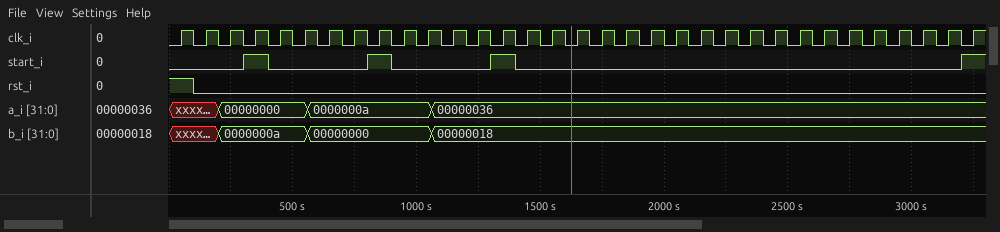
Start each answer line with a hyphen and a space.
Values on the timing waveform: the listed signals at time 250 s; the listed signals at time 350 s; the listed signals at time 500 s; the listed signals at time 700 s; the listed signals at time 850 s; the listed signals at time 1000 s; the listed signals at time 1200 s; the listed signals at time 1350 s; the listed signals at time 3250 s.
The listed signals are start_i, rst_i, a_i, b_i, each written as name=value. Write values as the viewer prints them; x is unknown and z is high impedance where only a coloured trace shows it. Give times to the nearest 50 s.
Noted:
- start_i=0, rst_i=0, a_i=00000000, b_i=0000000a
- start_i=1, rst_i=0, a_i=00000000, b_i=0000000a
- start_i=0, rst_i=0, a_i=00000000, b_i=0000000a
- start_i=0, rst_i=0, a_i=0000000a, b_i=00000000
- start_i=1, rst_i=0, a_i=0000000a, b_i=00000000
- start_i=0, rst_i=0, a_i=0000000a, b_i=00000000
- start_i=0, rst_i=0, a_i=00000036, b_i=00000018
- start_i=1, rst_i=0, a_i=00000036, b_i=00000018
- start_i=1, rst_i=0, a_i=00000036, b_i=00000018
